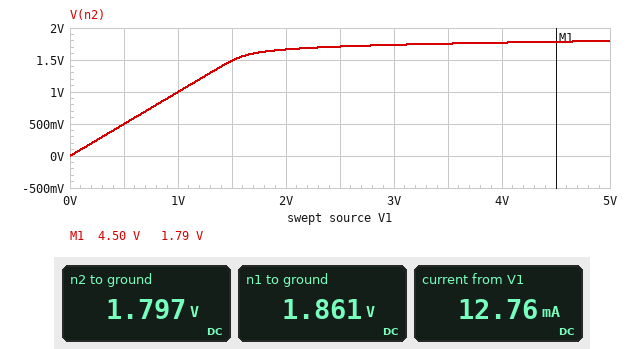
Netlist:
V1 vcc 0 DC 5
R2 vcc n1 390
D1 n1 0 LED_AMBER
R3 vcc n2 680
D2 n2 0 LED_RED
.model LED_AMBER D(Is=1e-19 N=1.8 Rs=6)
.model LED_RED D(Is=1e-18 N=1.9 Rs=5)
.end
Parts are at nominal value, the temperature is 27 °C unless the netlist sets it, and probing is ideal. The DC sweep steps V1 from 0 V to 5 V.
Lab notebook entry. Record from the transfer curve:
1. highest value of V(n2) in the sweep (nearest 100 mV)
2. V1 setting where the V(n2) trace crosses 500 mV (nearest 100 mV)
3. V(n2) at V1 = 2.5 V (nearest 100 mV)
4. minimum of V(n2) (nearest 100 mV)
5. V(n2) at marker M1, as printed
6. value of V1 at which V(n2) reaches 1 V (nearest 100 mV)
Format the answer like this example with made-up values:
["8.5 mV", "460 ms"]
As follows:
["1.8 V", "500 mV", "1.7 V", "0 V", "1.79 V", "1.0 V"]
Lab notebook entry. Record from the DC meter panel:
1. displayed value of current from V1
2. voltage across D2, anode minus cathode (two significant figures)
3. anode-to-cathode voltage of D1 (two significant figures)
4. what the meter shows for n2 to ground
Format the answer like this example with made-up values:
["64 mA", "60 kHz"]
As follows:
["12.76 mA", "1.8 V", "1.9 V", "1.797 V"]
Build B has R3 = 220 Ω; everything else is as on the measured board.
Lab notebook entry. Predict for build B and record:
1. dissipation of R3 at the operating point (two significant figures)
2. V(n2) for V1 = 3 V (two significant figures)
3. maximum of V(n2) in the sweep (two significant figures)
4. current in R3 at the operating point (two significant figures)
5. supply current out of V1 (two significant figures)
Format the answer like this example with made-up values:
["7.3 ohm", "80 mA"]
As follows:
["44 mW", "1.8 V", "1.9 V", "14 mA", "22 mA"]
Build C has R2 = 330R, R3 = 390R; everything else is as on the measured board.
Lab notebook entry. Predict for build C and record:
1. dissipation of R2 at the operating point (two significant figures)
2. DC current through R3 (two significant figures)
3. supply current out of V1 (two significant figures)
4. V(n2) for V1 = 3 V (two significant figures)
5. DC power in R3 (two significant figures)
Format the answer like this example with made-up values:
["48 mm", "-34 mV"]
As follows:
["30 mW", "8.1 mA", "18 mA", "1.8 V", "26 mW"]
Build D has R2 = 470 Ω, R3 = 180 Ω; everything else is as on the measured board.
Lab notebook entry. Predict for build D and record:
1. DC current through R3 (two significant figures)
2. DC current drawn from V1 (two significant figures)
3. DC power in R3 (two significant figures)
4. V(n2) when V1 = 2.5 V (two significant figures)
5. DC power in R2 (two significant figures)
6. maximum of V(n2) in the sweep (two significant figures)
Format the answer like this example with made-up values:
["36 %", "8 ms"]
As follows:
["17 mA", "24 mA", "53 mW", "1.8 V", "21 mW", "1.9 V"]
